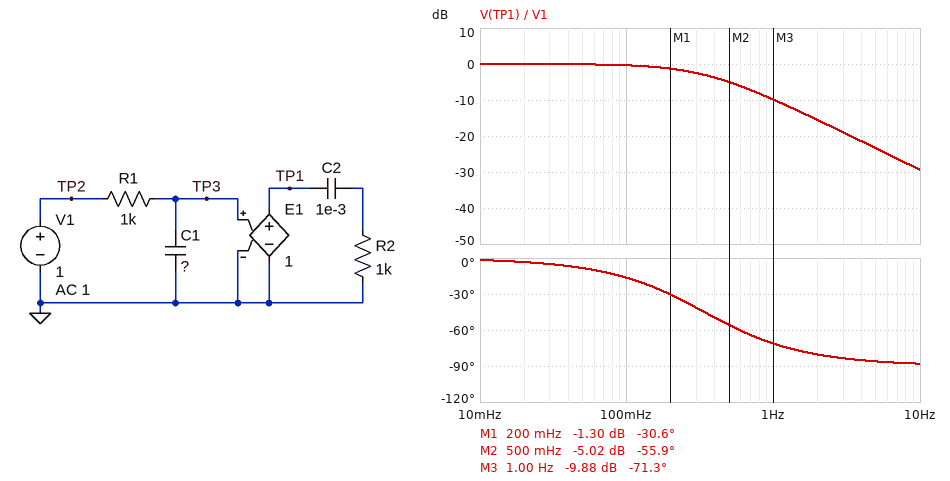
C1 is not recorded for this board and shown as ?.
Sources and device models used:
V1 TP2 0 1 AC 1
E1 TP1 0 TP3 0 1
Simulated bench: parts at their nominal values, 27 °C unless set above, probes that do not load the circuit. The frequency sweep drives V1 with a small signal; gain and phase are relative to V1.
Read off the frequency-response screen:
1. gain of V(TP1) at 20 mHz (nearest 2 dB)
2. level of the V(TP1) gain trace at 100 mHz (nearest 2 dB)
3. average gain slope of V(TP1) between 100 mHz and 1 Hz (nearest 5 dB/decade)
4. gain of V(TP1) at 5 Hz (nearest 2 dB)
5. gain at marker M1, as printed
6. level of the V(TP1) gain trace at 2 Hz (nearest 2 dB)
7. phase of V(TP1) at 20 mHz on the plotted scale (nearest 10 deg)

0 dB
0 dB
-10 dB/decade
-24 dB
-1.30 dB
-16 dB
0 deg
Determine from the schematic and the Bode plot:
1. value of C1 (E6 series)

470 µF
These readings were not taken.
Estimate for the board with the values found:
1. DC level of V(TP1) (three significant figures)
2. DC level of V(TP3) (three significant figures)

1.00 V
1.00 V
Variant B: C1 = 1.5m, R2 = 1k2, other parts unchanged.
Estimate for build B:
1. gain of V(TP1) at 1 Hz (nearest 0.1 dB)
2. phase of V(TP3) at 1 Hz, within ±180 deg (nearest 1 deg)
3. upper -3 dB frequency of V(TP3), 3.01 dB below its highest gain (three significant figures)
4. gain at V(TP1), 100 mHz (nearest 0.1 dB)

-19.5 dB
-84 deg
106 mHz
-2.8 dB
